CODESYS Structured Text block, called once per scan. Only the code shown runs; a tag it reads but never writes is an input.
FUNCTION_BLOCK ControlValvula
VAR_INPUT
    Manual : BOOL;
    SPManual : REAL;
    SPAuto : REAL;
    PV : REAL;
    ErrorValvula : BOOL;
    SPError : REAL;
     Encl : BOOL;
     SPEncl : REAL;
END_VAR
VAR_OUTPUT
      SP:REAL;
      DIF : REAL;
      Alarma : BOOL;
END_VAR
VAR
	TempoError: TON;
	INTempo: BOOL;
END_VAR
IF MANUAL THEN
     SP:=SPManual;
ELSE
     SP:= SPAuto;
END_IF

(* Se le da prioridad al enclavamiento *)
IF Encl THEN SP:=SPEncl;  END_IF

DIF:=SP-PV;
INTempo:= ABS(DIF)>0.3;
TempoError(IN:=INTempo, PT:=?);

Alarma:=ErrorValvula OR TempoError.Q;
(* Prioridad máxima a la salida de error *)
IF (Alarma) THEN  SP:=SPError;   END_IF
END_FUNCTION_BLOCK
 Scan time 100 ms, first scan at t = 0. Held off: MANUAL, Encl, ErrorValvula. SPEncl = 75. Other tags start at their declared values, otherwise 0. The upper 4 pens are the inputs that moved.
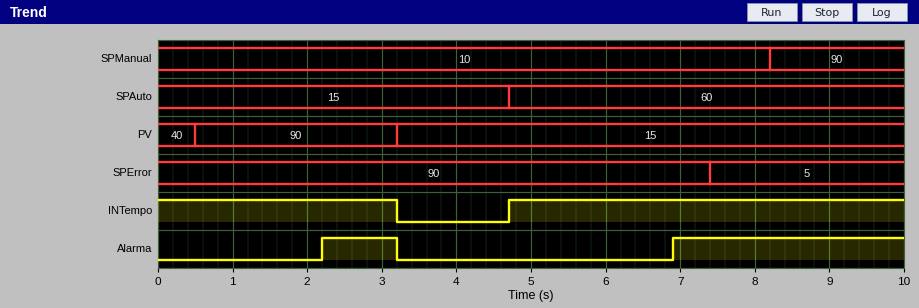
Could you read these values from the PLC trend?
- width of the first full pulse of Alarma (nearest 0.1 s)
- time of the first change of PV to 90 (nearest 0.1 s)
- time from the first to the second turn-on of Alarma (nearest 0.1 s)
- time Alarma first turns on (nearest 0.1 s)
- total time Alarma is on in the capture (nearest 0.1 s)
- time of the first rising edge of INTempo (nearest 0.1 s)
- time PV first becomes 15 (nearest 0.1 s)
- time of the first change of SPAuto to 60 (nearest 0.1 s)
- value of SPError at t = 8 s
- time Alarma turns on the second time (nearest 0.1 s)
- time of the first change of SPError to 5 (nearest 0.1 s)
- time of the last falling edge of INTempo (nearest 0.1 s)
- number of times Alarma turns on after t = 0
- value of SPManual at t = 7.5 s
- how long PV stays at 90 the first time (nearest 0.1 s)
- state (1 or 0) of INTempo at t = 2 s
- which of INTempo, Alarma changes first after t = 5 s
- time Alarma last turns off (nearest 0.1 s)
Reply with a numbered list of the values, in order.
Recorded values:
1. 1.0 s
2. 0.5 s
3. 4.7 s
4. 2.2 s
5. 4.1 s
6. 4.7 s
7. 3.2 s
8. 4.7 s
9. 5
10. 6.9 s
11. 7.4 s
12. 3.2 s
13. 2
14. 10
15. 2.7 s
16. 1
17. Alarma
18. 3.2 s
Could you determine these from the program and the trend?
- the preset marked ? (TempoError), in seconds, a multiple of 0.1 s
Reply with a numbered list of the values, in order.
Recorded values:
1. 2.2 s
